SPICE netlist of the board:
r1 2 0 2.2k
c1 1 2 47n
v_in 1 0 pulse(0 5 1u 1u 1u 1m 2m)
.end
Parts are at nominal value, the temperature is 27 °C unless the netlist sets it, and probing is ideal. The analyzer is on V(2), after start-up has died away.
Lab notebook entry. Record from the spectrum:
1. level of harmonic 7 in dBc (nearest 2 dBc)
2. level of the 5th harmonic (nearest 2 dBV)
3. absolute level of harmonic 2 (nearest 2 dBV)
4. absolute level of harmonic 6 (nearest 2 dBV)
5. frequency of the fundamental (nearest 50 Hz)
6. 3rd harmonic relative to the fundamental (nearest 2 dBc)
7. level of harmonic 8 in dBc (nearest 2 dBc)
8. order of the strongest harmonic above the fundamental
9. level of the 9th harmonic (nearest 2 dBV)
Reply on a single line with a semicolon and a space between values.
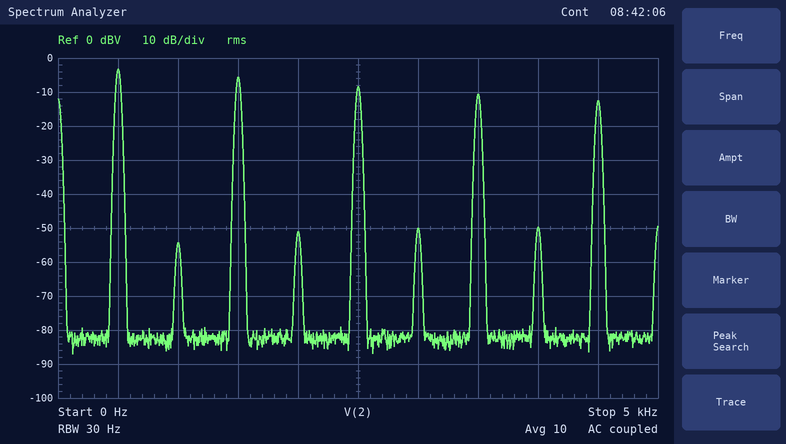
-8 dBc; -8 dBV; -54 dBV; -50 dBV; 500 Hz; -2 dBc; -46 dBc; 3; -12 dBV
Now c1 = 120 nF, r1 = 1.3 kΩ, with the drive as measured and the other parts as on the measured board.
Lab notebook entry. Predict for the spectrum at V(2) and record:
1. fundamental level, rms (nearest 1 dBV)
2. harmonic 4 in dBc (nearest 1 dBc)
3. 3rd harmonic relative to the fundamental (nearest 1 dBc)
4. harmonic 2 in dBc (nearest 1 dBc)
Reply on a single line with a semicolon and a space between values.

0 dBV; -50 dBc; -4 dBc; -52 dBc
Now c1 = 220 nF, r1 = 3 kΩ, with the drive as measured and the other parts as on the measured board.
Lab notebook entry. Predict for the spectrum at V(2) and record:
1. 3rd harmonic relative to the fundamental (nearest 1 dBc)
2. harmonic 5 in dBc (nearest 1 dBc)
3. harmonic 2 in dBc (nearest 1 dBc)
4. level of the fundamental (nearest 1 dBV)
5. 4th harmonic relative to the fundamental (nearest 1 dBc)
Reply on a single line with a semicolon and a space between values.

-9 dBc; -13 dBc; -55 dBc; 6 dBV; -55 dBc
